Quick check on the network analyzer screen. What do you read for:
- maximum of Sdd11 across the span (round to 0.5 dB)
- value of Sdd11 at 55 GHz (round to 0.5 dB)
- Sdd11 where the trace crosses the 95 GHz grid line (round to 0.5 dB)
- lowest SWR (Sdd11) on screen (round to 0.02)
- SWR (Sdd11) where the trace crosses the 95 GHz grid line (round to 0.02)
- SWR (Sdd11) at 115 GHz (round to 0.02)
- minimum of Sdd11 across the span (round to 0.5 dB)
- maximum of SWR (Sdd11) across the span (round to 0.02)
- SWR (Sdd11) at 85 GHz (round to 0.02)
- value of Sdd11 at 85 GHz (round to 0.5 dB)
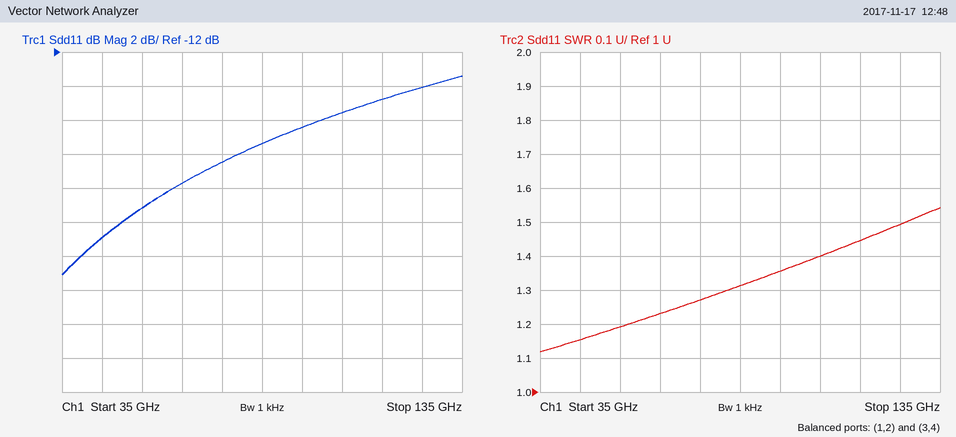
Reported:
-13.5 dB
-21.0 dB
-16.5 dB
1.12
1.36
1.44
-25.0 dB
1.54
1.32
-17.5 dB
